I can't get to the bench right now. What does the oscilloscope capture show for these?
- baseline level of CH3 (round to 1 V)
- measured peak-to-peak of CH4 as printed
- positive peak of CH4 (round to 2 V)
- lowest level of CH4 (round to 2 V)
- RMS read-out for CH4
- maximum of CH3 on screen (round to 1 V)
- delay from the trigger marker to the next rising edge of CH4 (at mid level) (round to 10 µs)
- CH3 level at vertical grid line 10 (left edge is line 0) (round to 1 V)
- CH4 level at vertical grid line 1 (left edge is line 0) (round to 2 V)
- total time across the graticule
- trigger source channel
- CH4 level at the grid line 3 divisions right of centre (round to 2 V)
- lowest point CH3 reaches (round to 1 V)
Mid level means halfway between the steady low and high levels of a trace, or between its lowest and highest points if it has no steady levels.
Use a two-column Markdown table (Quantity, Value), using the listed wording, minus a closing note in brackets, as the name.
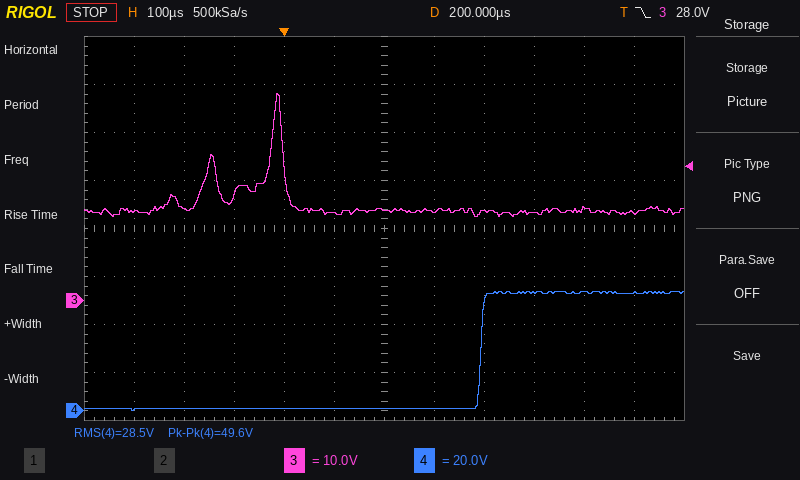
| Quantity | Value |
|---|---|
| baseline level of CH3 | 19 V |
| measured peak-to-peak of CH4 as printed | 49.6 V |
| positive peak of CH4 | 50 V |
| lowest level of CH4 | 0 V |
| RMS read-out for CH4 | 28.5 V |
| maximum of CH3 on screen | 43 V |
| delay from the trigger marker to the next rising edge of CH4 (at mid level) | 390 µs |
| CH3 level at vertical grid line 10 (left edge is line 0) | 19 V |
| CH4 level at vertical grid line 1 (left edge is line 0) | 0 V |
| total time across the graticule | 1.2 ms |
| trigger source channel | CH3 |
| CH4 level at the grid line 3 divisions right of centre | 50 V |
| lowest point CH3 reaches | 18 V |
